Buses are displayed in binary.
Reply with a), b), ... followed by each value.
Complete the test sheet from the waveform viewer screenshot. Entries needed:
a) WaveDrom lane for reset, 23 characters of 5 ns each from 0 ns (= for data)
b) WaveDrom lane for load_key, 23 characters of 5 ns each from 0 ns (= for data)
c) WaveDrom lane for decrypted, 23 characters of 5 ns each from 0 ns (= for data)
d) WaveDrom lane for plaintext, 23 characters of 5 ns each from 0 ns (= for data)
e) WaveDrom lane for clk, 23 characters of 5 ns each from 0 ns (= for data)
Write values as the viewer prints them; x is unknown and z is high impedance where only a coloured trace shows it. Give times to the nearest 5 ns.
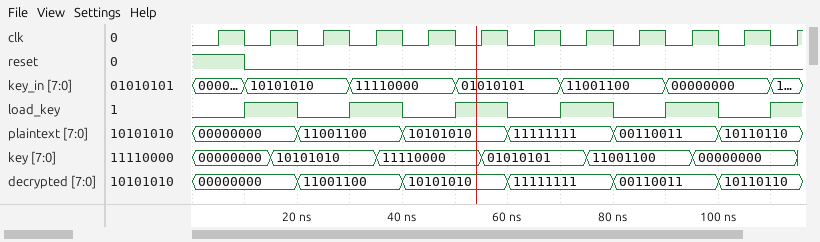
a) {name: 'reset', wave: '1.0....................'}
b) {name: 'load_key', wave: '0.1.0.1.0.1.0.1.0.1.0.1'}
c) {name: 'decrypted', wave: '=...=...=...=...=...=..', data: '00000000 11001100 10101010 11111111 00110011 10110110'}
d) {name: 'plaintext', wave: '=...=...=...=...=...=..', data: '00000000 11001100 10101010 11111111 00110011 10110110'}
e) {name: 'clk', wave: '01010101010101010101010'}
